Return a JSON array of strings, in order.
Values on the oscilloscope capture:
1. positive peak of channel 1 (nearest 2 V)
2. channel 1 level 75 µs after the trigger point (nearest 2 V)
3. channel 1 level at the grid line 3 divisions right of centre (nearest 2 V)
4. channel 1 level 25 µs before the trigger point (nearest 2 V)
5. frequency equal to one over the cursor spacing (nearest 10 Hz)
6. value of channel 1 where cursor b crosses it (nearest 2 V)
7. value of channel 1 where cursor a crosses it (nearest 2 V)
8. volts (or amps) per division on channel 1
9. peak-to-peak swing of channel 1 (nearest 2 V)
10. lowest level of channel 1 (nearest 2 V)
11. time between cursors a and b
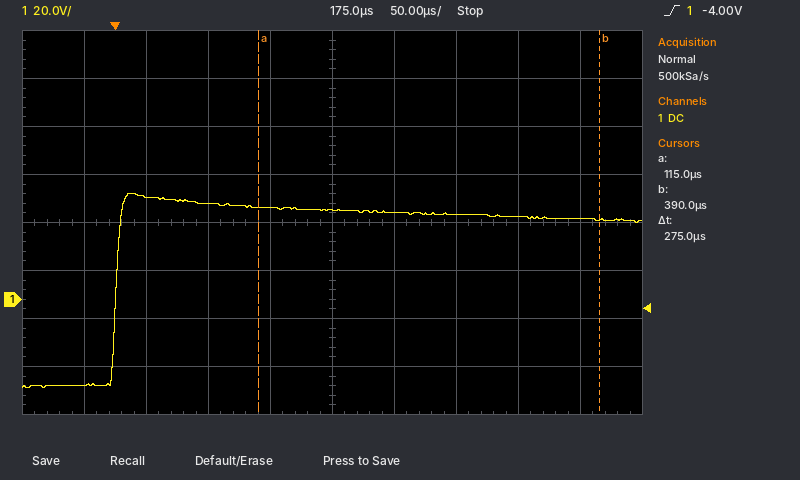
["44 V", "40 V", "34 V", "-36 V", "3.64 kHz", "34 V", "38 V", "20 V", "80 V", "-36 V", "275 µs"]
